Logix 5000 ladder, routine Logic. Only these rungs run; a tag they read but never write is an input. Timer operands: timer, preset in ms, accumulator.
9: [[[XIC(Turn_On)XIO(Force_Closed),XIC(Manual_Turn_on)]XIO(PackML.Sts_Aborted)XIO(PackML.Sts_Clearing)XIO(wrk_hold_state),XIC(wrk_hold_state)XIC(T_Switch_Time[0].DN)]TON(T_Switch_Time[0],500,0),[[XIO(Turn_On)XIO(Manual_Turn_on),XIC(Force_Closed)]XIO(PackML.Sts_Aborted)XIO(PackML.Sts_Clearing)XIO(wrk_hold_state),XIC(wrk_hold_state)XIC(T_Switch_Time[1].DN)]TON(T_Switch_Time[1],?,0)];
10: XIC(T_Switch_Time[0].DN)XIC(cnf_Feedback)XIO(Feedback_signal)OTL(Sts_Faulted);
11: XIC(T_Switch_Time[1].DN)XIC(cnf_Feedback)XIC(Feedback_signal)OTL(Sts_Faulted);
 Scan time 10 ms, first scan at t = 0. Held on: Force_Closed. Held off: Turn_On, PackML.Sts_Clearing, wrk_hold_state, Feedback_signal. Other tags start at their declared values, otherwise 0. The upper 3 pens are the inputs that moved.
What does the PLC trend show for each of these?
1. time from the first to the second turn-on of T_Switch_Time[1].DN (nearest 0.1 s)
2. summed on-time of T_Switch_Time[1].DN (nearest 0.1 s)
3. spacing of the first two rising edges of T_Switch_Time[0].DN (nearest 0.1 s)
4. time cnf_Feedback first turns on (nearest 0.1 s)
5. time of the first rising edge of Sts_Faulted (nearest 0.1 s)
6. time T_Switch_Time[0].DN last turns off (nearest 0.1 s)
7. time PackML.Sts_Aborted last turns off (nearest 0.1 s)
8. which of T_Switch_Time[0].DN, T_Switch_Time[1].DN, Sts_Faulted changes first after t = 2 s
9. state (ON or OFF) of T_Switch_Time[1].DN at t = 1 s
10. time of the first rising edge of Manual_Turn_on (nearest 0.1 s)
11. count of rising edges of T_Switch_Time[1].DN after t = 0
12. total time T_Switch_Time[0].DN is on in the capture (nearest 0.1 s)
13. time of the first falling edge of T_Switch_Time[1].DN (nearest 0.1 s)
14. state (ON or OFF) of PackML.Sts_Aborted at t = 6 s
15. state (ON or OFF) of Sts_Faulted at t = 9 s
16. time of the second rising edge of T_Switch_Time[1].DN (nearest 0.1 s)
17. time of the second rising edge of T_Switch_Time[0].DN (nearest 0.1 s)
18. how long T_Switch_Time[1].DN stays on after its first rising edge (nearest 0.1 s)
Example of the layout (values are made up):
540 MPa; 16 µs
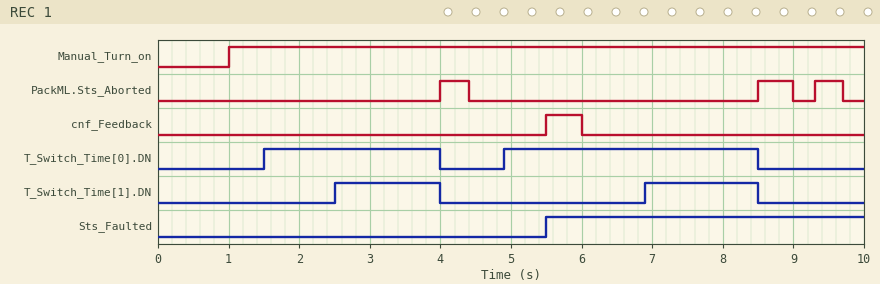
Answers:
4.4 s; 3.1 s; 3.4 s; 5.5 s; 5.5 s; 8.5 s; 9.7 s; T_Switch_Time[1].DN; OFF; 1.0 s; 2; 6.1 s; 4.0 s; OFF; ON; 6.9 s; 4.9 s; 1.5 s
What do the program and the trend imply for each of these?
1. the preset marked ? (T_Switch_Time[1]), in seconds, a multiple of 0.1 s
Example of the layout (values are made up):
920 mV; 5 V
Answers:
2.5 s
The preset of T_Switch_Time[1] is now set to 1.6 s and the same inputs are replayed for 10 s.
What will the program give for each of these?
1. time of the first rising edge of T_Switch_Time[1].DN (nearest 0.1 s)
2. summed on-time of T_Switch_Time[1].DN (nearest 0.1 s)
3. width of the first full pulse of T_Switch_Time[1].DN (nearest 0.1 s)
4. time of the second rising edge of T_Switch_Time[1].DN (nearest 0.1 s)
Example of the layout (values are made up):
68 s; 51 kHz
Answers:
1.6 s; 4.9 s; 2.4 s; 6.0 s
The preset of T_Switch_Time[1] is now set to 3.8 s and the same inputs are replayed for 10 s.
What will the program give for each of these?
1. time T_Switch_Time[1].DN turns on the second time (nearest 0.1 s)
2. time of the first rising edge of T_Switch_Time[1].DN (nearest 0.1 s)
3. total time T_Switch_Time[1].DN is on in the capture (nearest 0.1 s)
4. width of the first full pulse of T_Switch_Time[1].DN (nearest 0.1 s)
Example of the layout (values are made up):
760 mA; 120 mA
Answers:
8.2 s; 3.8 s; 0.5 s; 0.2 s
